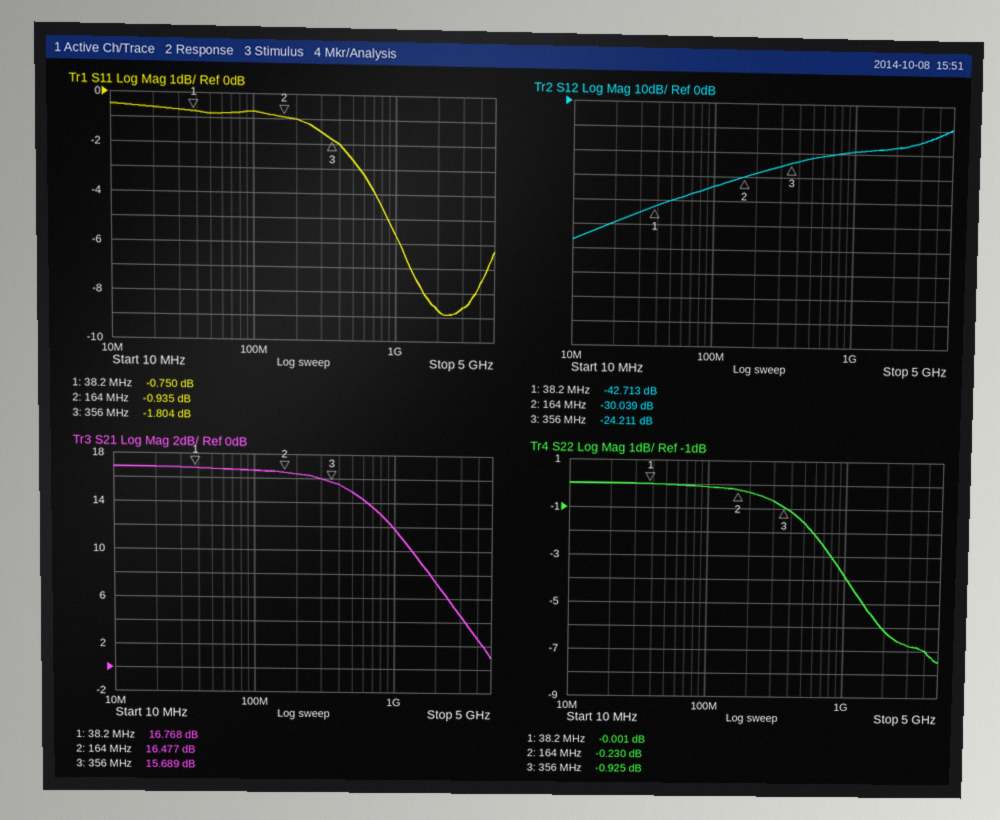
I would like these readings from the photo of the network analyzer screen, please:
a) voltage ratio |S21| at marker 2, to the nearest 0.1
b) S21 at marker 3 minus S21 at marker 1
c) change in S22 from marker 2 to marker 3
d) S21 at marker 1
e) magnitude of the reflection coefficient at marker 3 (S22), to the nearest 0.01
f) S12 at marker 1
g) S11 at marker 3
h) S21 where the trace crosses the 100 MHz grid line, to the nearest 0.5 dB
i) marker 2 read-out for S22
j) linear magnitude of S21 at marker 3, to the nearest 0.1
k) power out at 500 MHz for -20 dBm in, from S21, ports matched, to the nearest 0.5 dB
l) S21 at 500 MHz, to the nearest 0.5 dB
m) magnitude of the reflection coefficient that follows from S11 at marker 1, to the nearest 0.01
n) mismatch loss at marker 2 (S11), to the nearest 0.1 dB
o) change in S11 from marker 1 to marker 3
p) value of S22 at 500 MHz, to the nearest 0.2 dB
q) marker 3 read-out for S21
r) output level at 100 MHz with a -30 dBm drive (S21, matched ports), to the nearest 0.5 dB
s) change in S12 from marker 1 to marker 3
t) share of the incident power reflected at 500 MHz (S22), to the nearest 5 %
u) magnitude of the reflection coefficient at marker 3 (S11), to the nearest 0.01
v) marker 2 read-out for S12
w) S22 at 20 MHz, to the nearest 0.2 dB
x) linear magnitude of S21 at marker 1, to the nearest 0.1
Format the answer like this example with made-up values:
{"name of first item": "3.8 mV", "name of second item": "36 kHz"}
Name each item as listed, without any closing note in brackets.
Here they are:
{"voltage ratio |S21| at marker 2, to the nearest 0.1": "6.7", "S21 at marker 3 minus S21 at marker 1": "-1.079 dB", "change in S22 from marker 2 to marker 3": "-0.695 dB", "S21 at marker 1": "16.768 dB", "magnitude of the reflection coefficient at marker 3 (S22), to the nearest 0.01": "0.90", "S12 at marker 1": "-42.713 dB", "S11 at marker 3": "-1.804 dB", "S21 where the trace crosses the 100 MHz grid line, to the nearest 0.5 dB": "16.5 dB", "marker 2 read-out for S22": "-0.230 dB", "linear magnitude of S21 at marker 3, to the nearest 0.1": "6.1", "power out at 500 MHz for -20 dBm in, from S21, ports matched, to the nearest 0.5 dB": "-5.0 dBm", "S21 at 500 MHz, to the nearest 0.5 dB": "15.0 dB", "magnitude of the reflection coefficient that follows from S11 at marker 1, to the nearest 0.01": "0.92", "mismatch loss at marker 2 (S11), to the nearest 0.1 dB": "7.1 dB", "change in S11 from marker 1 to marker 3": "-1.054 dB", "value of S22 at 500 MHz, to the nearest 0.2 dB": "-1.6 dB", "marker 3 read-out for S21": "15.689 dB", "output level at 100 MHz with a -30 dBm drive (S21, matched ports), to the nearest 0.5 dB": "-13.5 dBm", "change in S12 from marker 1 to marker 3": "18.502 dB", "share of the incident power reflected at 500 MHz (S22), to the nearest 5 %": "70 %", "magnitude of the reflection coefficient at marker 3 (S11), to the nearest 0.01": "0.81", "marker 2 read-out for S12": "-30.039 dB", "S22 at 20 MHz, to the nearest 0.2 dB": "0.0 dB", "linear magnitude of S21 at marker 1, to the nearest 0.1": "6.9"}
